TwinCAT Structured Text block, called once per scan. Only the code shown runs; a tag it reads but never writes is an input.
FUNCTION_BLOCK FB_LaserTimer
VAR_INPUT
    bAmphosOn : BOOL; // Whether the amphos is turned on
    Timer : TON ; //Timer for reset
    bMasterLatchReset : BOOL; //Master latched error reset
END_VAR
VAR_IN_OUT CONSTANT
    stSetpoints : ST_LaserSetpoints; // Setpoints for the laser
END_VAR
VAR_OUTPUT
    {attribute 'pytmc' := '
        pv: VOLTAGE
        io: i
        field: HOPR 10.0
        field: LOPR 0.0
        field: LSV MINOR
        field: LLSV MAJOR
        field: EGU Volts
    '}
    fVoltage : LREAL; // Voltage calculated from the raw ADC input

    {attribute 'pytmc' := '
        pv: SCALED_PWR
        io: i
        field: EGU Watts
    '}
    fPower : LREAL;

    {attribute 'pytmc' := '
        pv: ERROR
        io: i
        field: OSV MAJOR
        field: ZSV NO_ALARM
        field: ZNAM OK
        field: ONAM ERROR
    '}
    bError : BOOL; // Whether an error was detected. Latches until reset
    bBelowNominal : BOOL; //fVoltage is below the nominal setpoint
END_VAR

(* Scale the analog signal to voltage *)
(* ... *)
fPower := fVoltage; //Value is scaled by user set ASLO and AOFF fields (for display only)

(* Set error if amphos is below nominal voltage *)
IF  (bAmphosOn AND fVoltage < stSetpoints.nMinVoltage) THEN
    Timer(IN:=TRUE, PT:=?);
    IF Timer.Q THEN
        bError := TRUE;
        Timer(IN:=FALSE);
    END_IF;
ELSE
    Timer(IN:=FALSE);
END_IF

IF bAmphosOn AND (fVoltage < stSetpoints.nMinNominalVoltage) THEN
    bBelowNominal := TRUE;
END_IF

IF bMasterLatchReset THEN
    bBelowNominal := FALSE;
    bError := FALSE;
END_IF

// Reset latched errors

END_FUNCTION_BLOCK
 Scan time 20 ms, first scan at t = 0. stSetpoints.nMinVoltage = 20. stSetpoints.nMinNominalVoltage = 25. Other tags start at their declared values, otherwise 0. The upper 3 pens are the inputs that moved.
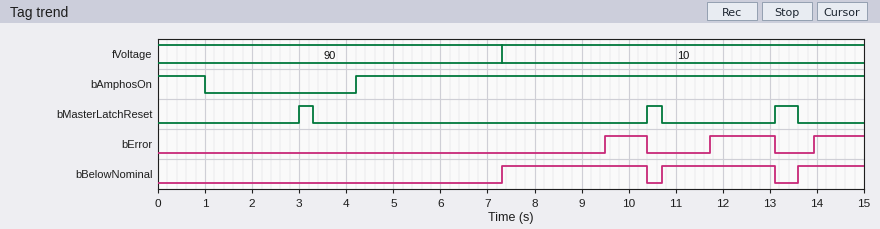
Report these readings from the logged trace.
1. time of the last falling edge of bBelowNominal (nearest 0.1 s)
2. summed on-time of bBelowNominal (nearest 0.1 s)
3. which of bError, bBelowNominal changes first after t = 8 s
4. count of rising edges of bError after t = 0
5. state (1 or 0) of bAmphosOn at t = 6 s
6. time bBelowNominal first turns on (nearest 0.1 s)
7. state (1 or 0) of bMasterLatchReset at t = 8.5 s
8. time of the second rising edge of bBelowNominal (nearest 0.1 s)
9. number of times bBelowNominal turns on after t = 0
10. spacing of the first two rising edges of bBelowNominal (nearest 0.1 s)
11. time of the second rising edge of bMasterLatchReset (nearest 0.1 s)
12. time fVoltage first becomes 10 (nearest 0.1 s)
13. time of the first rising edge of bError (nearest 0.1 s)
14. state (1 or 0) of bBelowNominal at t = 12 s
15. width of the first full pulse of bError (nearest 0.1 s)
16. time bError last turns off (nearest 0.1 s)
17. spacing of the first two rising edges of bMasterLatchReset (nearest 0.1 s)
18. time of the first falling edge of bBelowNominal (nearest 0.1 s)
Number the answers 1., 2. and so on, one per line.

1. 13.1 s
2. 6.9 s
3. bError
4. 3
5. 1
6. 7.3 s
7. 0
8. 10.7 s
9. 3
10. 3.4 s
11. 10.4 s
12. 7.3 s
13. 9.5 s
14. 1
15. 0.9 s
16. 13.1 s
17. 7.4 s
18. 10.4 s
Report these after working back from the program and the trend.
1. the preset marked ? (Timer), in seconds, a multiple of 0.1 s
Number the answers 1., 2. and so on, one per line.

1. 2.2 s
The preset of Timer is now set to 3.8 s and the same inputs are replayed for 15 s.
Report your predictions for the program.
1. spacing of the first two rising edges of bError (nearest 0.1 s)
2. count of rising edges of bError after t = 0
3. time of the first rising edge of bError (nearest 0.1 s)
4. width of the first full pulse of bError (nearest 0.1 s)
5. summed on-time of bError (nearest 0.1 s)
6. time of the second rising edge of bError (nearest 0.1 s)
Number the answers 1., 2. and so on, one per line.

1. 3.8 s
2. 2
3. 11.1 s
4. 2.0 s
5. 2.1 s
6. 14.9 s
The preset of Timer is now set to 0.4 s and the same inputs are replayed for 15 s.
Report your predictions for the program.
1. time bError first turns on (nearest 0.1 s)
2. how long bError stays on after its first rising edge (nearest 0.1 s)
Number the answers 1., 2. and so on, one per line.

1. 7.7 s
2. 2.7 s
